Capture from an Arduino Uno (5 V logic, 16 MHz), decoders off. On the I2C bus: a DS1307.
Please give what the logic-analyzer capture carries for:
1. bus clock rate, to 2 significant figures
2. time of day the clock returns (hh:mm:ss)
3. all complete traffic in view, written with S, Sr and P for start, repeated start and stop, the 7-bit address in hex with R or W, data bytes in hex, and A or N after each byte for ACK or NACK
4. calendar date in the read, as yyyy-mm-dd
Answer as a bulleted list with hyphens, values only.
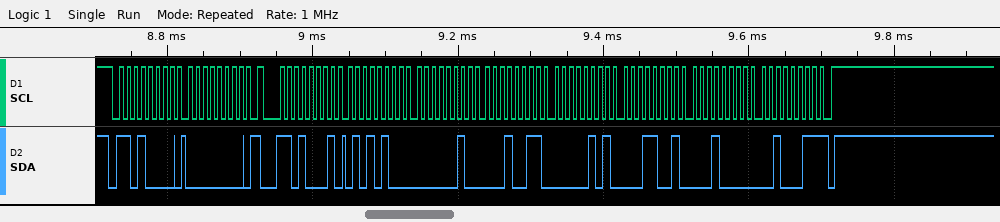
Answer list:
- 100 kHz
- 13:02:54
- S 68W A 00 A Sr 68R A 54 A 02 A 13 A 05 A 19 A 10 A 23 N P
- 2023-10-19
